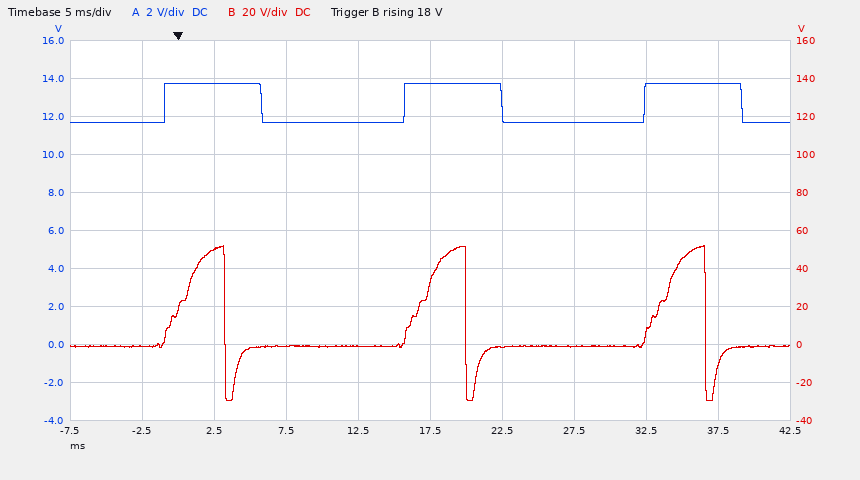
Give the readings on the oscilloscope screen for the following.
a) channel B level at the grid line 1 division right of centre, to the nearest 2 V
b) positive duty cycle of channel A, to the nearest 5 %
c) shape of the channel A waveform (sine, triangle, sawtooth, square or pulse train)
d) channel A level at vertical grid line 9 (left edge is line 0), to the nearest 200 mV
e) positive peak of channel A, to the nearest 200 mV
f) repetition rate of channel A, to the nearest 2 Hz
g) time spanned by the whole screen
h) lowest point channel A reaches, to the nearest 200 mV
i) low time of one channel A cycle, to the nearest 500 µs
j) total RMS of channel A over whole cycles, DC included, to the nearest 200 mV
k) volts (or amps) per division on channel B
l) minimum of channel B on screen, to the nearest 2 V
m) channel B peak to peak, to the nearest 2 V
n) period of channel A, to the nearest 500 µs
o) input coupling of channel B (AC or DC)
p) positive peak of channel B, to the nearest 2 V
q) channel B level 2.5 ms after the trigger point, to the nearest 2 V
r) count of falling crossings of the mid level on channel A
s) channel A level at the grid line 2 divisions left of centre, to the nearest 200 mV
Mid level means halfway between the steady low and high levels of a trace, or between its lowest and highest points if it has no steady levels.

-2 V
40 %
pulse train
13.8 V
13.8 V
60 Hz
50 ms
11.6 V
10.0 ms
12.6 V
20 V
-30 V
82 V
16.5 ms
DC
52 V
50 V
3
11.6 V
